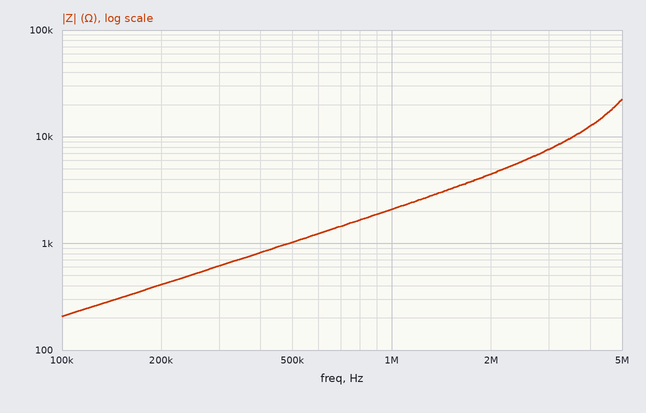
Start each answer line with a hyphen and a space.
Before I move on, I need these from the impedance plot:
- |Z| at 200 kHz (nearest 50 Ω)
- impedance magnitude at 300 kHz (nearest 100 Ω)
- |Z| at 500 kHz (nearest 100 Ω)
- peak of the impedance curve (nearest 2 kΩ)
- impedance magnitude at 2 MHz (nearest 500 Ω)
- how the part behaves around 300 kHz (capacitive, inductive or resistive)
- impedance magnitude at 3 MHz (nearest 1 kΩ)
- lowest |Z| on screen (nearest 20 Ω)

- 400 Ω
- 600 Ω
- 1.0 kΩ
- 22 kΩ
- 4.5 kΩ
- inductive
- 8 kΩ
- 200 Ω
